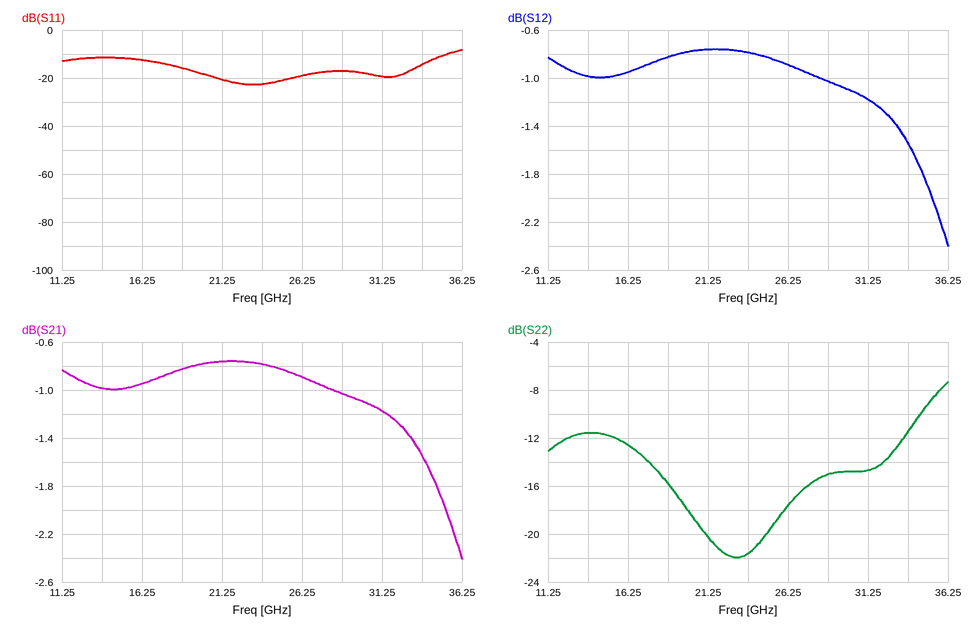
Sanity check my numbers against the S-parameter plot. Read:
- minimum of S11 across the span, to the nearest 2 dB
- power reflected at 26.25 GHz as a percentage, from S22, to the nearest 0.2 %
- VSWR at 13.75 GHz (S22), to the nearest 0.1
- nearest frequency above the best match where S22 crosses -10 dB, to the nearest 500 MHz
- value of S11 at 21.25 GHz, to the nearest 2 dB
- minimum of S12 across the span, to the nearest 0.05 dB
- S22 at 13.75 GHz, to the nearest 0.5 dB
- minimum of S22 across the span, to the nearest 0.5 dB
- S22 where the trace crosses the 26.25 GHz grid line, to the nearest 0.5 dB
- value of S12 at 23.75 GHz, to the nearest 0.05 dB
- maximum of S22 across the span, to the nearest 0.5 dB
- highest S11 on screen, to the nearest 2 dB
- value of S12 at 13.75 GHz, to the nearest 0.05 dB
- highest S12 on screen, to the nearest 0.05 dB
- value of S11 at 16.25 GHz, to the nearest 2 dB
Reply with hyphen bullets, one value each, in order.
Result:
- -22 dB
- 1.8 %
- 1.7
- 34.5 GHz
- -20 dB
- -2.40 dB
- -11.5 dB
- -22.0 dB
- -17.5 dB
- -0.80 dB
- -7.5 dB
- -8 dB
- -1.00 dB
- -0.75 dB
- -12 dB
